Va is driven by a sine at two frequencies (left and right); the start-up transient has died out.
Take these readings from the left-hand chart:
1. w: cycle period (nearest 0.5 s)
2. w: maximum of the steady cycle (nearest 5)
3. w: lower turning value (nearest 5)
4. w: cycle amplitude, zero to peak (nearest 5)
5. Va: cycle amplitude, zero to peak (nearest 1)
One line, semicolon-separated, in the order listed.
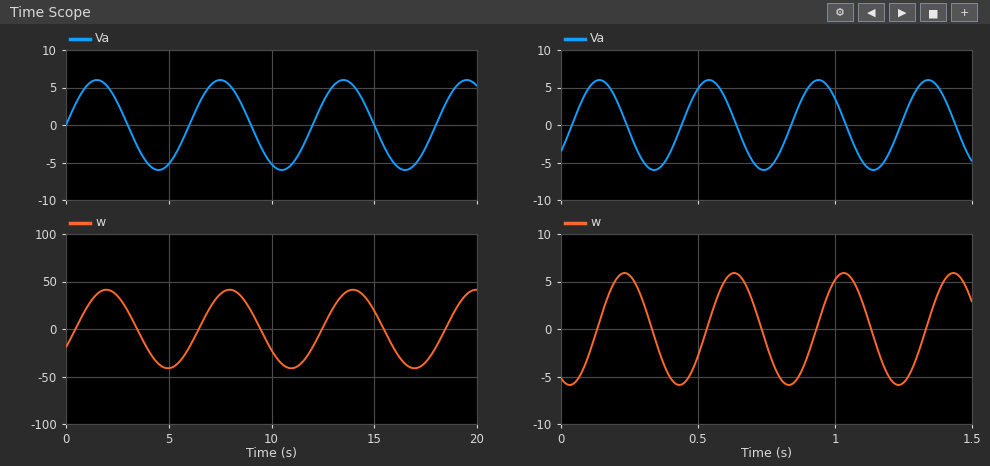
6.0 s; 40; -40; 40; 6
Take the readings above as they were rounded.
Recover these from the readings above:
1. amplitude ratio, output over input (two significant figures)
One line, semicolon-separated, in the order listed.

6.7
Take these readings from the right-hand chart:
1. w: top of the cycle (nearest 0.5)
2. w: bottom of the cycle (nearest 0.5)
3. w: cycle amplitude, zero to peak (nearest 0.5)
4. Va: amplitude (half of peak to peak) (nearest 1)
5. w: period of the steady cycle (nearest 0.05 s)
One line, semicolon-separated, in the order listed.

6.0; -6.0; 6.0; 6; 0.40 s
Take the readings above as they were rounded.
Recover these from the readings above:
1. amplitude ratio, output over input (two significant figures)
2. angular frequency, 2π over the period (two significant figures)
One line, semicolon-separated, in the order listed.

1.0; 16 rad/s
